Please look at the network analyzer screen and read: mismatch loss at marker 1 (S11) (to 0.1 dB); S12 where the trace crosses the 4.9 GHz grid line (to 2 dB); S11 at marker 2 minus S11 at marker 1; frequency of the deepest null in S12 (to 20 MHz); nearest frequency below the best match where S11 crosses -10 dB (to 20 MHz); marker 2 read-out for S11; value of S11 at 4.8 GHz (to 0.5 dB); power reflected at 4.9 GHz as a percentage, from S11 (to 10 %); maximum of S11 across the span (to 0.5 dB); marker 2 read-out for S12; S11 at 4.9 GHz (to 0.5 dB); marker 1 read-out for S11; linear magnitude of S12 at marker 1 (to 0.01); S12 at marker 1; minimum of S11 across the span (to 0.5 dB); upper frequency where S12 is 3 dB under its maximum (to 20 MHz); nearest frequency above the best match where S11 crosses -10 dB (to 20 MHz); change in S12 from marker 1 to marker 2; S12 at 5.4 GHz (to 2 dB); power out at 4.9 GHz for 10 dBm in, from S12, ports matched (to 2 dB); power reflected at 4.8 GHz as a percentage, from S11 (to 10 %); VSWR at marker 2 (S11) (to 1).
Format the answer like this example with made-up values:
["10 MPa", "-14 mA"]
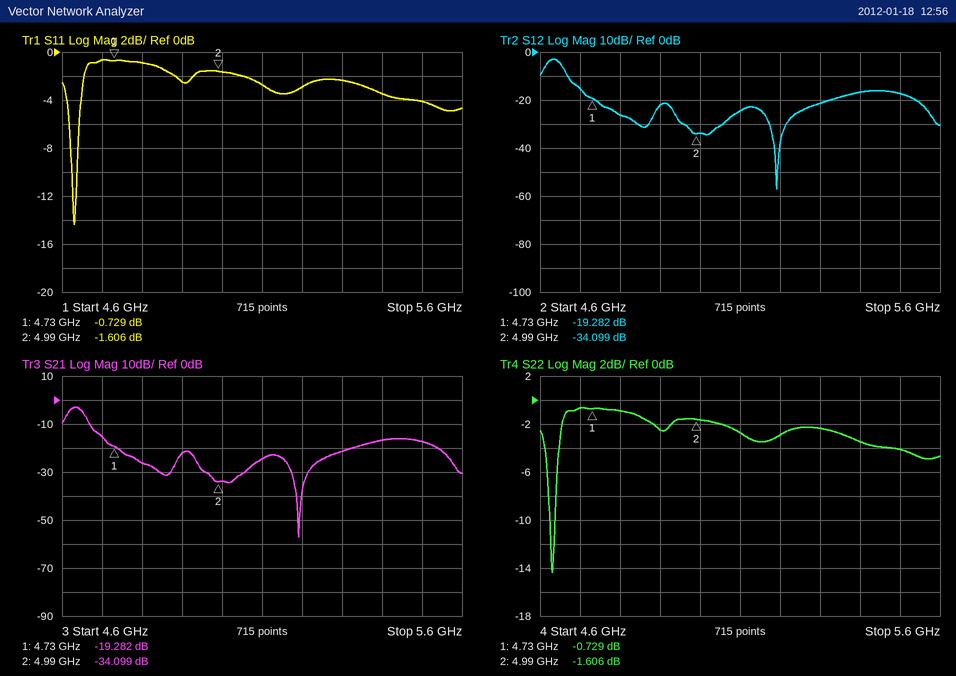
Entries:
["8.1 dB", "-22 dB", "-0.877 dB", "5.20 GHz", "4.62 GHz", "-1.606 dB", "-1.0 dB", "60 %", "-0.5 dB", "-34.099 dB", "-2.5 dB", "-0.729 dB", "0.11", "-19.282 dB", "-14.5 dB", "4.66 GHz", "4.64 GHz", "-14.817 dB", "-16 dB", "-12 dBm", "80 %", "11"]
